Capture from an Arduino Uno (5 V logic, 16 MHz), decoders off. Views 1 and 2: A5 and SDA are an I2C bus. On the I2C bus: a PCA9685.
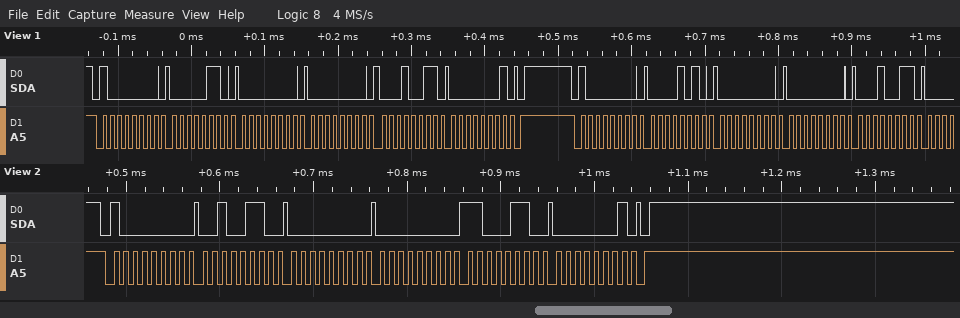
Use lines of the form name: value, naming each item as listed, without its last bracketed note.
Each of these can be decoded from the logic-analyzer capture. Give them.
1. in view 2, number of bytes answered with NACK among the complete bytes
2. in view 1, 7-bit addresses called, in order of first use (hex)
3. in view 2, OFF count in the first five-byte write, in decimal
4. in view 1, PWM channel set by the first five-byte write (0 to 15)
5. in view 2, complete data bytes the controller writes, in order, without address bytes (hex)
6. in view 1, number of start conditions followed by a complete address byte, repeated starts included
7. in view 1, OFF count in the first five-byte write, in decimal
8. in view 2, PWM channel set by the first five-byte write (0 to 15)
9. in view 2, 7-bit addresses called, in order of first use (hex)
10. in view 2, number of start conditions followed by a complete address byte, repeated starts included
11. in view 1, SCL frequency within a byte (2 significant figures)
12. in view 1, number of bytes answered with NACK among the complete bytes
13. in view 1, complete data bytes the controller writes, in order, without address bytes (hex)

in view 2, number of bytes answered with NACK among the complete bytes: 0
in view 1, 7-bit addresses called, in order of first use: 0x40
in view 2, OFF count in the first five-byte write, in decimal: 454
in view 1, PWM channel set by the first five-byte write: 0
in view 2, complete data bytes the controller writes, in order, without address bytes: 26 00 00 C6 01
in view 1, number of start conditions followed by a complete address byte, repeated starts included: 2
in view 1, OFF count in the first five-byte write, in decimal: 275
in view 2, PWM channel set by the first five-byte write: 8
in view 2, 7-bit addresses called, in order of first use: 0x40
in view 2, number of start conditions followed by a complete address byte, repeated starts included: 1
in view 1, SCL frequency within a byte: 100 kHz
in view 1, number of bytes answered with NACK among the complete bytes: 0
in view 1, complete data bytes the controller writes, in order, without address bytes: 06 00 00 13 01 0A 00 00 13
